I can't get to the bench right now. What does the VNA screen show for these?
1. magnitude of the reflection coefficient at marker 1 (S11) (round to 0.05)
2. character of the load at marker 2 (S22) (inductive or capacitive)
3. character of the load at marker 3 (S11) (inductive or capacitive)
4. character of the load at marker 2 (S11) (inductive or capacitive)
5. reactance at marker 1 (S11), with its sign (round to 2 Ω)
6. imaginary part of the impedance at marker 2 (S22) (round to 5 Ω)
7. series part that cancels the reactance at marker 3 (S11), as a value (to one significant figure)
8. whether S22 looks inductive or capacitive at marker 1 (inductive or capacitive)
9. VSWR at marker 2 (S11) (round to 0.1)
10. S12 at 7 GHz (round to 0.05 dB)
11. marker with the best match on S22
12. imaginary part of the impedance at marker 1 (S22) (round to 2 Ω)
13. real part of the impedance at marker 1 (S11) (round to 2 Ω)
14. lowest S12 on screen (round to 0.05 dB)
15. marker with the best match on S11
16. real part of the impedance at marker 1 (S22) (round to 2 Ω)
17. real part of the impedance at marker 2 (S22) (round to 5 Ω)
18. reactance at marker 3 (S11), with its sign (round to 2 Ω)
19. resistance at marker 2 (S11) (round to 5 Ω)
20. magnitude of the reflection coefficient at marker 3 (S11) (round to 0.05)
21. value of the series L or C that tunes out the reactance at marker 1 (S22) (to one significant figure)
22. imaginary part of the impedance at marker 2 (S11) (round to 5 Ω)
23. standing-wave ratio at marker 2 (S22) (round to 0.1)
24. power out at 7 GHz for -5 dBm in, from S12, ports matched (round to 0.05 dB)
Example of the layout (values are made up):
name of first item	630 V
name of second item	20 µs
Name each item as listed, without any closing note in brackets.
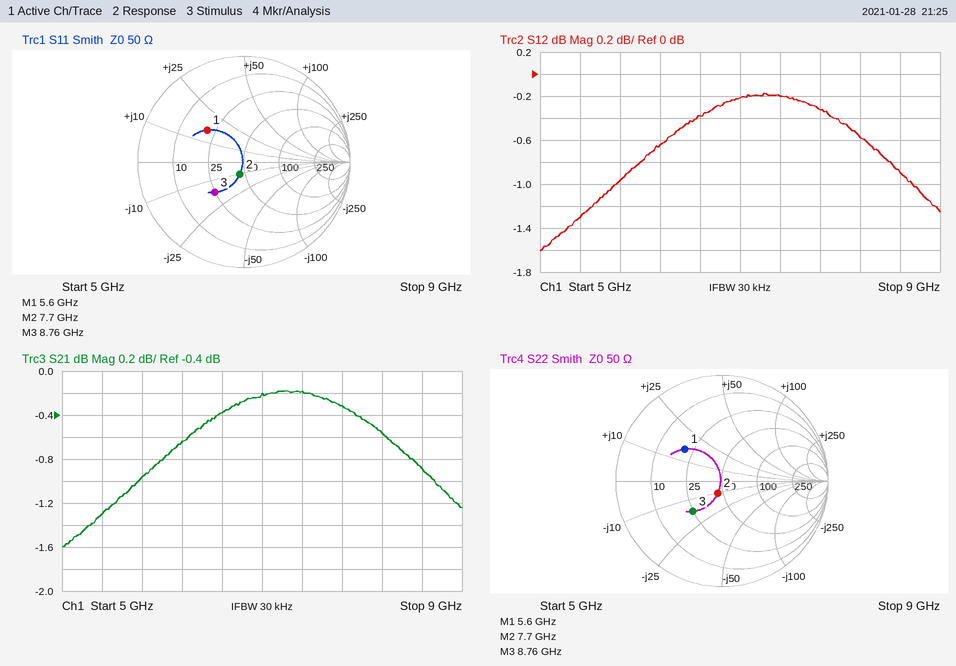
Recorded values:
magnitude of the reflection coefficient at marker 1 (S11)	0.45
character of the load at marker 2 (S22)	capacitive
character of the load at marker 3 (S11)	capacitive
character of the load at marker 2 (S11)	capacitive
reactance at marker 1 (S11), with its sign	+16 Ω
imaginary part of the impedance at marker 2 (S22)	-10 Ω
series part that cancels the reactance at marker 3 (S11), as a value	300 pH
whether S22 looks inductive or capacitive at marker 1	inductive
VSWR at marker 2 (S11)	1.3
S12 at 7 GHz	-0.20 dB
marker with the best match on S22	marker 2
imaginary part of the impedance at marker 1 (S22)	+16 Ω
real part of the impedance at marker 1 (S11)	20 Ω
lowest S12 on screen	-1.60 dB
marker with the best match on S11	marker 2
real part of the impedance at marker 1 (S22)	20 Ω
real part of the impedance at marker 2 (S22)	45 Ω
reactance at marker 3 (S11), with its sign	-16 Ω
resistance at marker 2 (S11)	45 Ω
magnitude of the reflection coefficient at marker 3 (S11)	0.40
value of the series L or C that tunes out the reactance at marker 1 (S22)	2 pF
imaginary part of the impedance at marker 2 (S11)	-10 Ω
standing-wave ratio at marker 2 (S22)	1.3
power out at 7 GHz for -5 dBm in, from S12, ports matched	-5.20 dBm
